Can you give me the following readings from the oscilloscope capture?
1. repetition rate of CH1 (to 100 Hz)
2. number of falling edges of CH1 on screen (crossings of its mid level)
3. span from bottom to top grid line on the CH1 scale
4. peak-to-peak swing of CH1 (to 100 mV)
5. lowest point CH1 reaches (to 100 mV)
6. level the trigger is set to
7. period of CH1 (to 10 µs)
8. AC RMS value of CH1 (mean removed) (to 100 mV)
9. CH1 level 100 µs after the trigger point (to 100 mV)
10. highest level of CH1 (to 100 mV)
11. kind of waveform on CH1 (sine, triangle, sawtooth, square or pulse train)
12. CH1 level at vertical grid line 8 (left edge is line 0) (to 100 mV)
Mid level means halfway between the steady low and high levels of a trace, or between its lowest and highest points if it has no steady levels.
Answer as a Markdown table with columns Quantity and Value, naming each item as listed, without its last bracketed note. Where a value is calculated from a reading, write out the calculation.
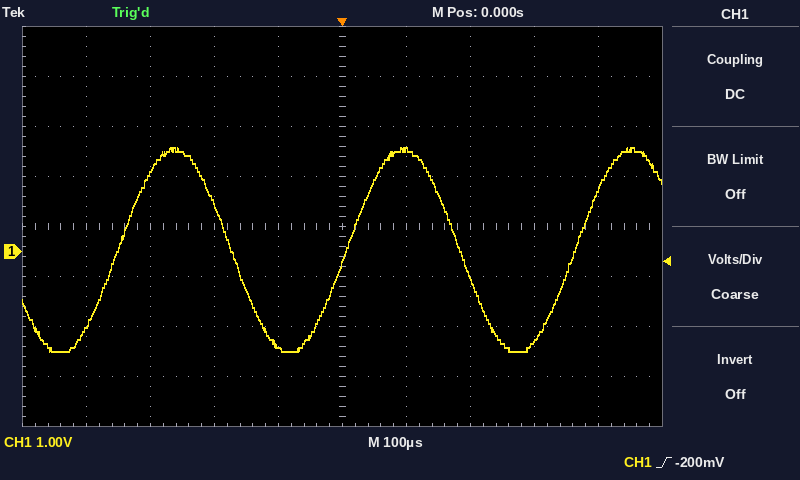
| Quantity | Value |
|---|---|
| repetition rate of CH1 | 1 / 360 µs ≈ 2.8 kHz |
| number of falling edges of CH1 on screen | 2 |
| span from bottom to top grid line on the CH1 scale | 8 V |
| peak-to-peak swing of CH1 | 2.1 V − (-2.0 V) = 4.1 V |
| lowest point CH1 reaches | -2.0 V |
| level the trigger is set to | -200 mV |
| period of CH1 | 360 µs |
| AC RMS value of CH1 (mean removed) | 4.1 V / (2√2) ≈ 1.4 V |
| CH1 level 100 µs after the trigger point | 2.0 V |
| highest level of CH1 | 2.1 V |
| kind of waveform on CH1 | sine |
| CH1 level at vertical grid line 8 (left edge is line 0) | -1.8 V |
